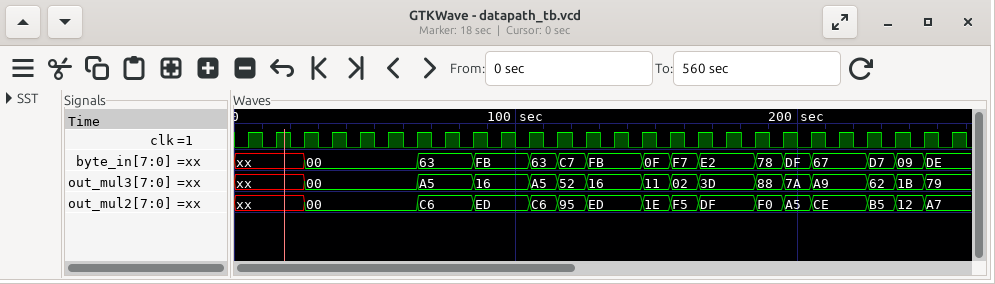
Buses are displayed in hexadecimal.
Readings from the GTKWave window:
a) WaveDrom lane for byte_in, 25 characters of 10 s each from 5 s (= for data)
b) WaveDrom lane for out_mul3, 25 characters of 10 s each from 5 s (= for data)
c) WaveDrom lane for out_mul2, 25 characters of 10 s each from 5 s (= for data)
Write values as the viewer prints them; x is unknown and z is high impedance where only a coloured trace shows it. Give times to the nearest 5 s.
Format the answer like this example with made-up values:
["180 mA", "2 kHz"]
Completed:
["{name: 'byte_in', wave: 'x.=...=.=.===.===.===.===', data: '00 63 FB 63 C7 FB 0F F7 E2 78 DF 67 D7 09 DE'}", "{name: 'out_mul3', wave: 'x.=...=.=.===.===.===.===', data: '00 A5 16 A5 52 16 11 02 3D 88 7A A9 62 1B 79'}", "{name: 'out_mul2', wave: 'x.=...=.=.===.===.===.===', data: '00 C6 ED C6 95 ED 1E F5 DF F0 A5 CE B5 12 A7'}"]
